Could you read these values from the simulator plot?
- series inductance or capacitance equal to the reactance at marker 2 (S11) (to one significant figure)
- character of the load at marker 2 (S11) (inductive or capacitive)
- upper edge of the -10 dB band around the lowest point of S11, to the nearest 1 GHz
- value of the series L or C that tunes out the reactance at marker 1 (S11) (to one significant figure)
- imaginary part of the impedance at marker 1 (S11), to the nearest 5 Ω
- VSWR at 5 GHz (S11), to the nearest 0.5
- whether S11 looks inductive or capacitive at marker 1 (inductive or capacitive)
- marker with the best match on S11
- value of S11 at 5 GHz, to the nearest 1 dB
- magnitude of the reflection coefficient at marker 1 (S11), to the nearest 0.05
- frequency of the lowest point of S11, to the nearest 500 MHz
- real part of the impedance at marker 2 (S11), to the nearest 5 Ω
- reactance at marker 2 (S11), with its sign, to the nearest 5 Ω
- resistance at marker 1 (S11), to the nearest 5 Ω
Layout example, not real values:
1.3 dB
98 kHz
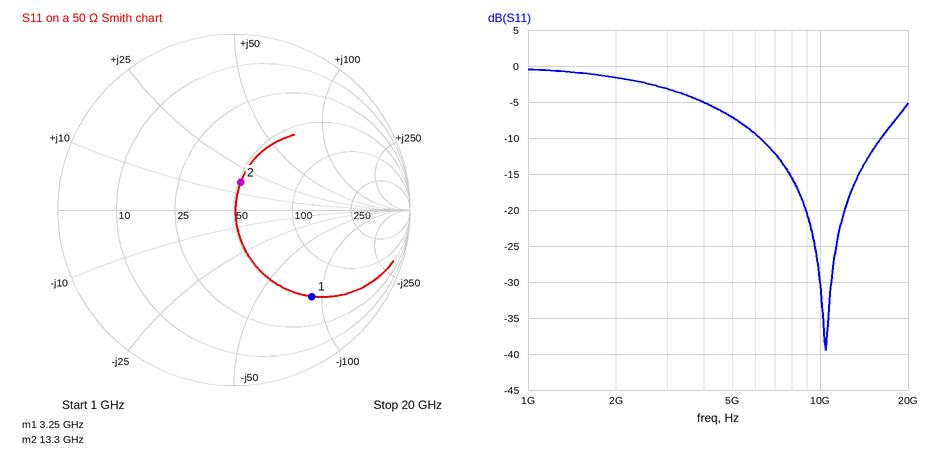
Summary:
200 pH
inductive
16 GHz
4 nH
-90 Ω
2.5
capacitive
marker 2
-7 dB
0.65
10.5 GHz
50 Ω
+15 Ω
50 Ω
